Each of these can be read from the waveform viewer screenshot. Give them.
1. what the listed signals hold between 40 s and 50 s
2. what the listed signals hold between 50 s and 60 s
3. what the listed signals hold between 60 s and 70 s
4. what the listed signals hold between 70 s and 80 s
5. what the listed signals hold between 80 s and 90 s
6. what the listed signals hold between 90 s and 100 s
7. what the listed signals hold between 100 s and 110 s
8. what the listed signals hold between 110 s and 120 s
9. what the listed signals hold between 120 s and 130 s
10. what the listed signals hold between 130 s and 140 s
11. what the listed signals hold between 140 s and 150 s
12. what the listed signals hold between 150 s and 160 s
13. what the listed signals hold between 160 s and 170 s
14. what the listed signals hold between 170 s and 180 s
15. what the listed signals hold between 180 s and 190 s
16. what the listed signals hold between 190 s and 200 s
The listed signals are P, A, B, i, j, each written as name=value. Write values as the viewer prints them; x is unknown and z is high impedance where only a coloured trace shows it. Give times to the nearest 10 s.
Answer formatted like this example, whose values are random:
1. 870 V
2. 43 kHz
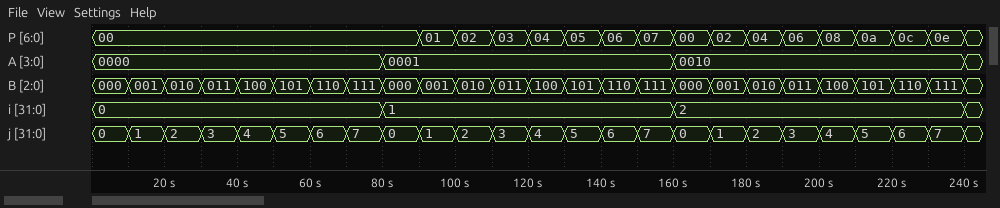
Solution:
1. P=00, A=0000, B=100, i=0, j=4
2. P=00, A=0000, B=101, i=0, j=5
3. P=00, A=0000, B=110, i=0, j=6
4. P=00, A=0000, B=111, i=0, j=7
5. P=00, A=0001, B=000, i=1, j=0
6. P=01, A=0001, B=001, i=1, j=1
7. P=02, A=0001, B=010, i=1, j=2
8. P=03, A=0001, B=011, i=1, j=3
9. P=04, A=0001, B=100, i=1, j=4
10. P=05, A=0001, B=101, i=1, j=5
11. P=06, A=0001, B=110, i=1, j=6
12. P=07, A=0001, B=111, i=1, j=7
13. P=00, A=0010, B=000, i=2, j=0
14. P=02, A=0010, B=001, i=2, j=1
15. P=04, A=0010, B=010, i=2, j=2
16. P=06, A=0010, B=011, i=2, j=3
